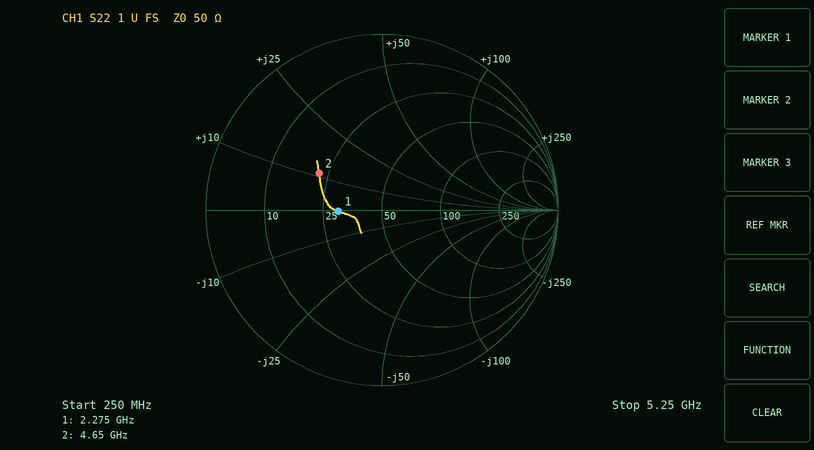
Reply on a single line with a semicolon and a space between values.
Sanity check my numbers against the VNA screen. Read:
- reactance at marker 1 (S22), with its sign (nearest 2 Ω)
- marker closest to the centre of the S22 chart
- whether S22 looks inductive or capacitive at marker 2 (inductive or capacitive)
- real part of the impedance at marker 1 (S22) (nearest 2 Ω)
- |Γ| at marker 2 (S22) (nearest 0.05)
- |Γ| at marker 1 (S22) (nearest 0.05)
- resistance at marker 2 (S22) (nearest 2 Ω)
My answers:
0 Ω; marker 1; inductive; 30 Ω; 0.40; 0.25; 22 Ω
